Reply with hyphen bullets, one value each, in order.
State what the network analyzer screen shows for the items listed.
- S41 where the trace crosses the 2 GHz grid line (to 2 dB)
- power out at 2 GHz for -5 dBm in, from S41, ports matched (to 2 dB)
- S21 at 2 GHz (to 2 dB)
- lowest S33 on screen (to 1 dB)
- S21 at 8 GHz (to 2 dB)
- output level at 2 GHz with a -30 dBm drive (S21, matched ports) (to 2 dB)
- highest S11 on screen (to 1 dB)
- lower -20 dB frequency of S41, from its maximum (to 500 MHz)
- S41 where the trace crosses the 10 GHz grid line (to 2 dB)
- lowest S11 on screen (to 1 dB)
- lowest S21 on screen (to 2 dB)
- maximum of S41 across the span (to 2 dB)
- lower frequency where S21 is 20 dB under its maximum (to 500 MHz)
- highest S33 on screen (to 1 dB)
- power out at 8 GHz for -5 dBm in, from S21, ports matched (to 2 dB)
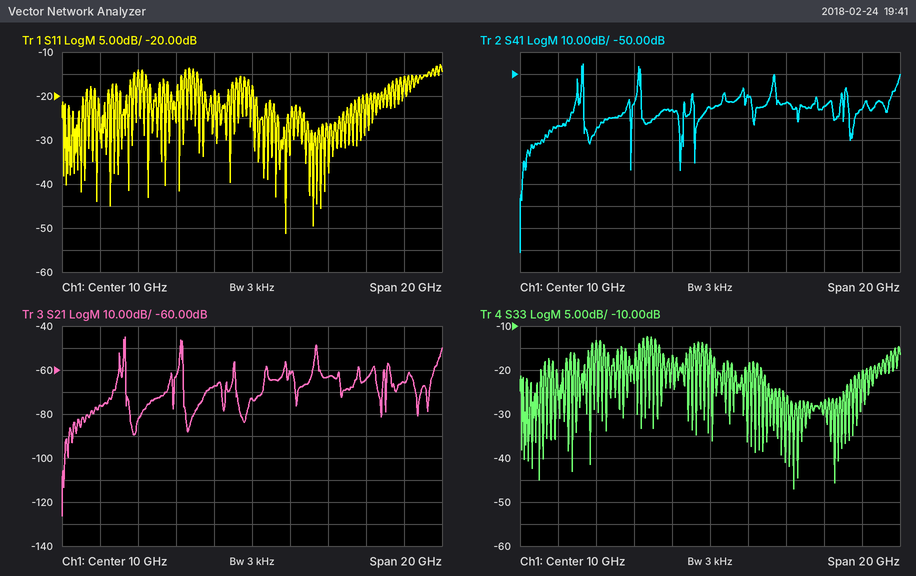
- -74 dB
- -78 dBm
- -76 dB
- -47 dB
- -68 dB
- -106 dBm
- -13 dB
- 3.0 GHz
- -66 dB
- -51 dB
- -126 dB
- -46 dB
- 3.0 GHz
- -12 dB
- -72 dBm
